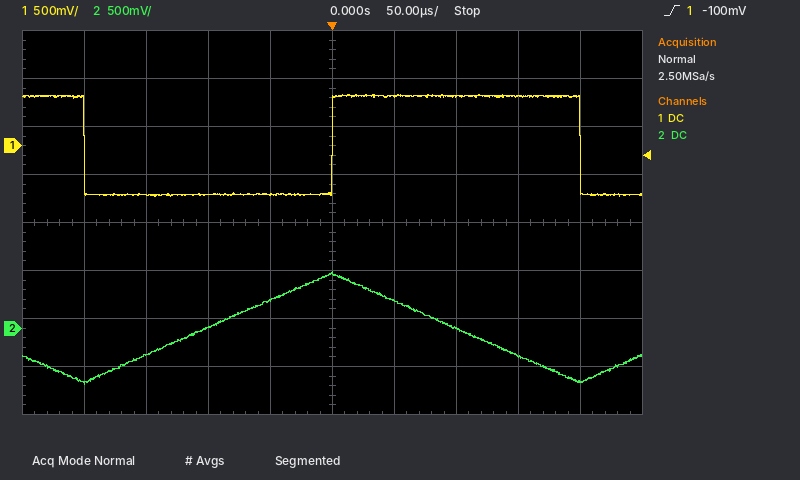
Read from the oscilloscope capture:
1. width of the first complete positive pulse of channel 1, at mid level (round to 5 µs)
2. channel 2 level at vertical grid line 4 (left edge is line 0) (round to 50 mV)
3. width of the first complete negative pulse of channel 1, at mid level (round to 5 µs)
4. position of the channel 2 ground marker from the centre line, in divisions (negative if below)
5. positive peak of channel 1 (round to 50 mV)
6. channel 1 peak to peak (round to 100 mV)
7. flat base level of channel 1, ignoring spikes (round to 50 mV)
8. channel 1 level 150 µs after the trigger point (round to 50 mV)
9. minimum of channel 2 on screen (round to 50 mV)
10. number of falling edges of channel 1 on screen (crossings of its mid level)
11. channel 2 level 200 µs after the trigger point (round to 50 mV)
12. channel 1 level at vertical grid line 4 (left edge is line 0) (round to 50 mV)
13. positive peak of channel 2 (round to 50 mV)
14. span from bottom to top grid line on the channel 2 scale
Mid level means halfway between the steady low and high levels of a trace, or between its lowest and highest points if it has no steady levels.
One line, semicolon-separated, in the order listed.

200 µs; 300 mV; 200 µs; -2.2 div; 550 mV; 1.10 V; -500 mV; 500 mV; -600 mV; 2; -550 mV; -500 mV; 600 mV; 4 V
